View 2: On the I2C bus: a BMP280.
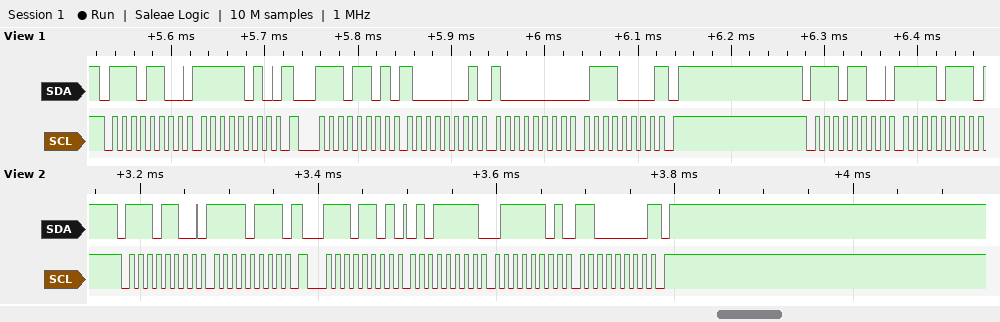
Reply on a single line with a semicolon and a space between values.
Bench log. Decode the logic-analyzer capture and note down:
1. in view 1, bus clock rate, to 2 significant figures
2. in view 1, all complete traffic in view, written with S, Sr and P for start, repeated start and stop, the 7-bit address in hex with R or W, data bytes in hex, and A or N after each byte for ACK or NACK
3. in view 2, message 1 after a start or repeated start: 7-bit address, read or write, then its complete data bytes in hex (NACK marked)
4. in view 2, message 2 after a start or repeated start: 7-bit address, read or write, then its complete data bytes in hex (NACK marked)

100 kHz; S 76W A FA A Sr 76R A 81 A 80 A 70 N P S 76W A F7 A; 0x76 write: F7; 0x76 read: 5F 7D C0 NACK
